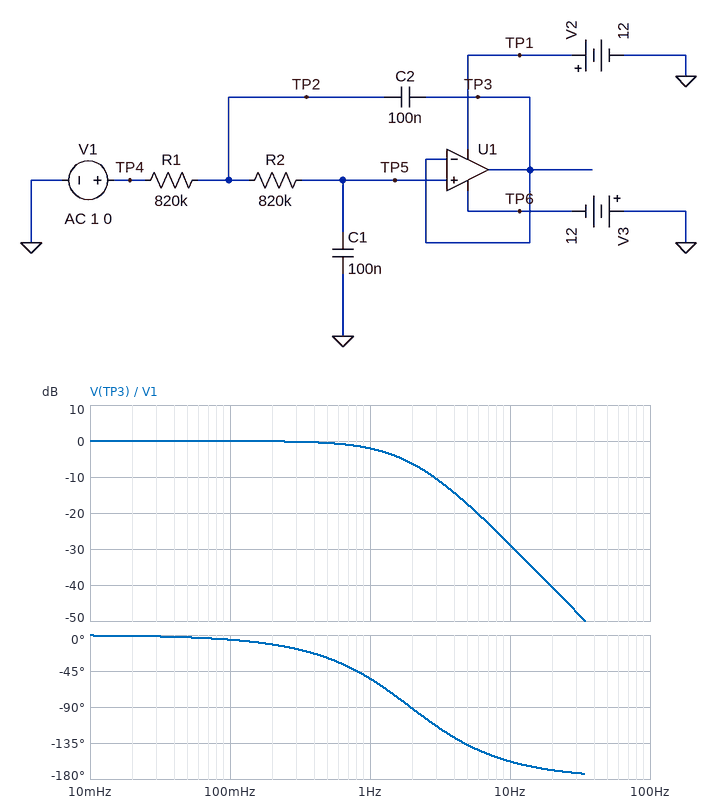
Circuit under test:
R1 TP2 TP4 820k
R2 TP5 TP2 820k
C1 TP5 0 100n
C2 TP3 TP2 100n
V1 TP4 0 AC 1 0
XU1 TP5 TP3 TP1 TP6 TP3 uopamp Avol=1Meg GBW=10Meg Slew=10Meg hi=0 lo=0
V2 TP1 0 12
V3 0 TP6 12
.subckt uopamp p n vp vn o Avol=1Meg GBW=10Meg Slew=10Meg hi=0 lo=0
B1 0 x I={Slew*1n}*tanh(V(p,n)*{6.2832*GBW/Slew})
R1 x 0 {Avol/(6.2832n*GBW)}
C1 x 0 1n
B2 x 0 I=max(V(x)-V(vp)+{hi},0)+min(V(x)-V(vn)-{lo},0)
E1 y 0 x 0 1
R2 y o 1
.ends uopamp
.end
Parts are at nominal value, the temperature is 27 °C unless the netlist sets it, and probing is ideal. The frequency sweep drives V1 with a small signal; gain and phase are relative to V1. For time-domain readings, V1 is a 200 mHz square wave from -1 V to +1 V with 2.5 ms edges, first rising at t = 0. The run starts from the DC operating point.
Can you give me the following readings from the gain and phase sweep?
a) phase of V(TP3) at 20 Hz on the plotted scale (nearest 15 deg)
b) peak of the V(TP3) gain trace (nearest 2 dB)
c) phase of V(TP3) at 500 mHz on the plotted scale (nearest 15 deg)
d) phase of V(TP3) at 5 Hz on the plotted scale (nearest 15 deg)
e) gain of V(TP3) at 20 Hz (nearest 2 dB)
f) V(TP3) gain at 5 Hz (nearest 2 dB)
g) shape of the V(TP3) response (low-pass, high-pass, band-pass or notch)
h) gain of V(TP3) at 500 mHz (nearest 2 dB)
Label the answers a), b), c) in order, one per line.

a) -165 deg
b) 0 dB
c) -30 deg
d) -135 deg
e) -40 dB
f) -18 dB
g) low-pass
h) 0 dB
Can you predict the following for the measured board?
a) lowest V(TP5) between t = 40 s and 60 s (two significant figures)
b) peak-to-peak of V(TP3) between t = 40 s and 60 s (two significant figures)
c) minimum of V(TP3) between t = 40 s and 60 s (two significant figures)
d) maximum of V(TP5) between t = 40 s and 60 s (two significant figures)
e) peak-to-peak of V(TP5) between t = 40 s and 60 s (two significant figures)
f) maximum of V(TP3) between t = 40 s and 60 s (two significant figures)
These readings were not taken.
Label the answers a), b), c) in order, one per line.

a) -1.0 V
b) 2.0 V
c) -1.0 V
d) 1.0 V
e) 2.0 V
f) 1.0 V
